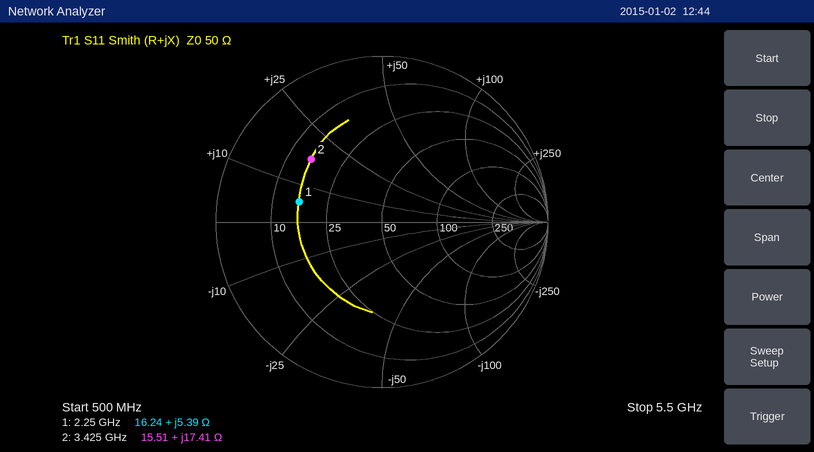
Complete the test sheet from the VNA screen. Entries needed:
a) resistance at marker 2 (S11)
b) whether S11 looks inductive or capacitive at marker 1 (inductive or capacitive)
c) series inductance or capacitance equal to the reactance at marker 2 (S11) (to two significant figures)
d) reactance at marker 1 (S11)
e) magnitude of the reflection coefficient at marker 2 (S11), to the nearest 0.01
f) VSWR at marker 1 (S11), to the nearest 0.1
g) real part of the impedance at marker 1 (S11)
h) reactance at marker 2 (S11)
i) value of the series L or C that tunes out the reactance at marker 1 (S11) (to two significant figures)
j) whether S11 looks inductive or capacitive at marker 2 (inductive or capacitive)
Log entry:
15.51 Ω
inductive
810 pH
+5.39 Ω
0.57
3.1
16.24 Ω
+17.41 Ω
13 pF
inductive
